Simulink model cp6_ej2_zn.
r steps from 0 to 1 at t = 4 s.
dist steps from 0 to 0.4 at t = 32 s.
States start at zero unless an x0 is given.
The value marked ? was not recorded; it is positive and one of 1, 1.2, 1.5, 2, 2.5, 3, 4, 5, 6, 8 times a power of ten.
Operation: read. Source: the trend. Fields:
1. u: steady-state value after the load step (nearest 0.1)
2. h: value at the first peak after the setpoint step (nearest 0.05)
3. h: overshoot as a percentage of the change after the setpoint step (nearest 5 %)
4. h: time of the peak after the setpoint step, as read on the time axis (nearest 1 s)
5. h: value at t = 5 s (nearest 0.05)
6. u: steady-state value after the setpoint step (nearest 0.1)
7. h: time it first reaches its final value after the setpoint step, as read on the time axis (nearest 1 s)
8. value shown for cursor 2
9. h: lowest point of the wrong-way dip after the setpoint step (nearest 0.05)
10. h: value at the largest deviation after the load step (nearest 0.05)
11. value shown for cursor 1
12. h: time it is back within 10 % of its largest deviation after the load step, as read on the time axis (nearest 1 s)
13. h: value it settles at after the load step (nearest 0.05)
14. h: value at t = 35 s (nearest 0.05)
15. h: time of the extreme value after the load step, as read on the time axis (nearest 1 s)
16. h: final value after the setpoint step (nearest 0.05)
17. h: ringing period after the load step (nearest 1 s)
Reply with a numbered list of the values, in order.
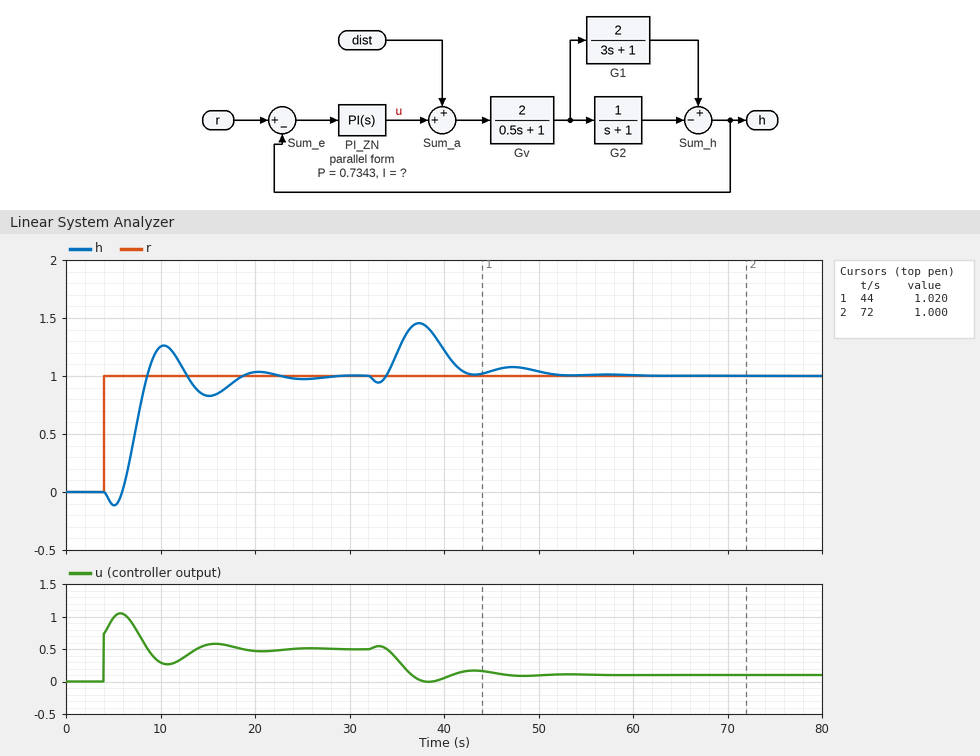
1. 0.1
2. 1.25
3. 25 %
4. 10 s
5. -0.10
6. 0.5
7. 9 s
8. 1.000
9. -0.10
10. 1.45
11. 1.020
12. 50 s
13. 1.00
14. 1.20
15. 37 s
16. 1.00
17. 10 s
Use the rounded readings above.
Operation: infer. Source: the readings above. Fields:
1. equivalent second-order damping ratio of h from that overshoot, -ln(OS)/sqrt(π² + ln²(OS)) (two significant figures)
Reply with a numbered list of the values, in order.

1. 0.40
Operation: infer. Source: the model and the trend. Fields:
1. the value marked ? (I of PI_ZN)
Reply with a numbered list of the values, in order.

1. 0.15
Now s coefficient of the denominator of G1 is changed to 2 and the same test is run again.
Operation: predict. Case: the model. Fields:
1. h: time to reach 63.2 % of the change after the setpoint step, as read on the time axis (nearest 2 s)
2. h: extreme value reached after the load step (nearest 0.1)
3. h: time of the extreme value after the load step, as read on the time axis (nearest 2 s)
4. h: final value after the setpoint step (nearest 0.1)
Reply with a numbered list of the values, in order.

1. 6 s
2. 1.3
3. 36 s
4. 1.0
